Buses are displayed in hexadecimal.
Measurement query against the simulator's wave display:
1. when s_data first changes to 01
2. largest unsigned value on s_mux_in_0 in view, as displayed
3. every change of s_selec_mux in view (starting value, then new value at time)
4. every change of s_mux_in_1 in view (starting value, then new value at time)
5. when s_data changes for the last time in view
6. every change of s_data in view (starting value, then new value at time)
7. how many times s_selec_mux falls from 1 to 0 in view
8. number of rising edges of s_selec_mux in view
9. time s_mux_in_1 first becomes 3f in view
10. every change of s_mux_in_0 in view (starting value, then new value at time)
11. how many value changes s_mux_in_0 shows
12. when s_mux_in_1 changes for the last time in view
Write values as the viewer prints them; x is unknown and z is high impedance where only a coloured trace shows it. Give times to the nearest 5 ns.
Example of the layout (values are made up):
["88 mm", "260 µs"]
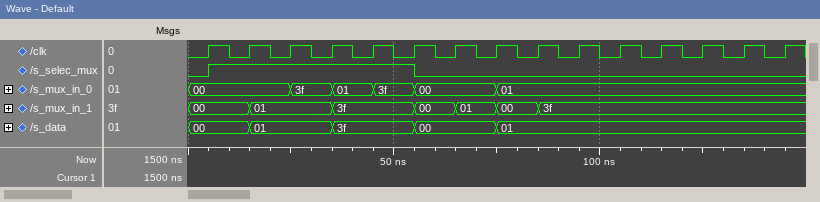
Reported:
["15 ns", "3f", "0, 1 at 5 ns, 0 at 55 ns", "00, 01 at 15 ns, 3f at 35 ns, 00 at 55 ns, 01 at 65 ns, 00 at 75 ns, 3f at 85 ns", "75 ns", "00, 01 at 15 ns, 3f at 35 ns, 00 at 55 ns, 01 at 75 ns", "1", "1", "35 ns", "00, 3f at 25 ns, 01 at 35 ns, 3f at 45 ns, 00 at 55 ns, 01 at 75 ns", "5", "85 ns"]
